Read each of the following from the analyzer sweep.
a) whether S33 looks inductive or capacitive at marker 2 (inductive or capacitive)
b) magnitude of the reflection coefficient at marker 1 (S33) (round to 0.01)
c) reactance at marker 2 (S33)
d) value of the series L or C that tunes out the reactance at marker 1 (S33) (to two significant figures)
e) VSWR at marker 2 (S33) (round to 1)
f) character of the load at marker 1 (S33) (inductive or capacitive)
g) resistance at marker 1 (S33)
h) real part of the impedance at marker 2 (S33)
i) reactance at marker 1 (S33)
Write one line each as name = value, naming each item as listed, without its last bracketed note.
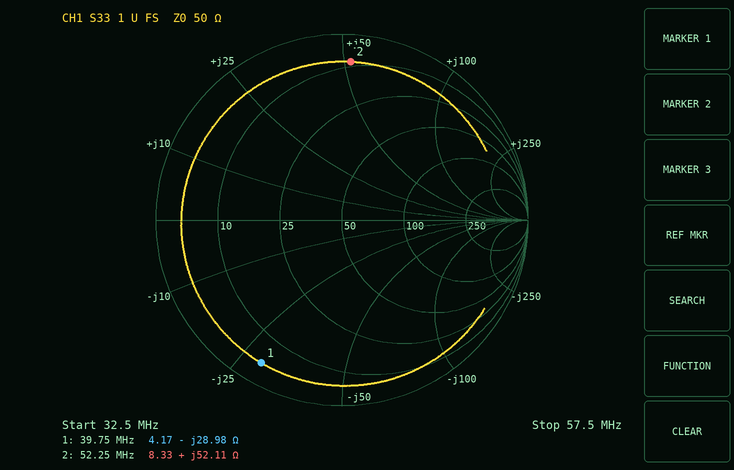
whether S33 looks inductive or capacitive at marker 2 = inductive
magnitude of the reflection coefficient at marker 1 (S33) = 0.88
reactance at marker 2 = +52.11 Ω
value of the series L or C that tunes out the reactance at marker 1 (S33) = 120 nH
VSWR at marker 2 (S33) = 13
character of the load at marker 1 (S33) = capacitive
resistance at marker 1 = 4.17 Ω
real part of the impedance at marker 2 = 8.33 Ω
reactance at marker 1 = -28.98 Ω
